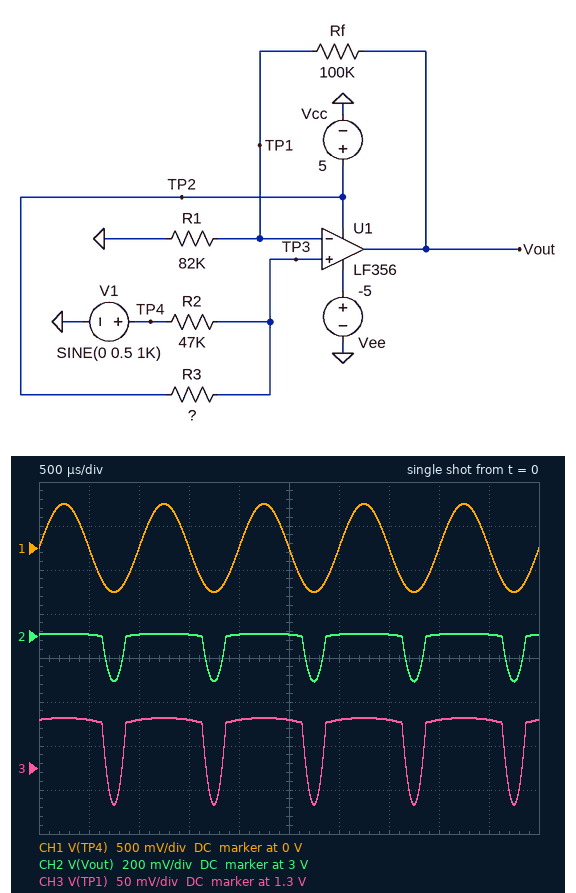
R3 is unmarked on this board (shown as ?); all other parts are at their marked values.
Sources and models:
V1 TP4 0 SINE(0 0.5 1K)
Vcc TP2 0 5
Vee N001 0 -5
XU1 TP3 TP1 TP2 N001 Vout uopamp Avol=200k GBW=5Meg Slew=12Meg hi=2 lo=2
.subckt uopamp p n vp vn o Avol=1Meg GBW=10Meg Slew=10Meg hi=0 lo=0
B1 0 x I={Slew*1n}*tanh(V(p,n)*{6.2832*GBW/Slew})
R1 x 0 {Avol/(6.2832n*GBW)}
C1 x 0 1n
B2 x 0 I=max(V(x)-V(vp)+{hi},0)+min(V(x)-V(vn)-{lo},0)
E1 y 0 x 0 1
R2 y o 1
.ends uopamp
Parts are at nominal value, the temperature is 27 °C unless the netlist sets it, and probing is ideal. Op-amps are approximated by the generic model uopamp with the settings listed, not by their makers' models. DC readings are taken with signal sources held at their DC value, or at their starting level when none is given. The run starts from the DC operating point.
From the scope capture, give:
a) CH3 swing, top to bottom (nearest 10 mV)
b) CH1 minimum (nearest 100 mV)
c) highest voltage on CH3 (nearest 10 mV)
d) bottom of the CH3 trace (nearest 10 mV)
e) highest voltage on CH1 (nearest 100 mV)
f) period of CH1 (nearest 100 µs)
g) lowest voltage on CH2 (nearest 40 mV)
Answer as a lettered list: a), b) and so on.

a) 100 mV
b) -500 mV
c) 1.36 V
d) 1.26 V
e) 500 mV
f) 1.0 ms
g) 2.80 V
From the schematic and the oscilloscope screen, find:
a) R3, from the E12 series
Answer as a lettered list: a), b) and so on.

a) 100 kΩ
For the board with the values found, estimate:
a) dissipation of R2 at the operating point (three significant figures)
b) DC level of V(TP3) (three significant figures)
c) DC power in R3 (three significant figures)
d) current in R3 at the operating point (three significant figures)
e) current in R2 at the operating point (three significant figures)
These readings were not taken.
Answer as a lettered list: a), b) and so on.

a) 54.4 µW
b) 1.60 V
c) 116 µW
d) 34.0 µA
e) 34.0 µA
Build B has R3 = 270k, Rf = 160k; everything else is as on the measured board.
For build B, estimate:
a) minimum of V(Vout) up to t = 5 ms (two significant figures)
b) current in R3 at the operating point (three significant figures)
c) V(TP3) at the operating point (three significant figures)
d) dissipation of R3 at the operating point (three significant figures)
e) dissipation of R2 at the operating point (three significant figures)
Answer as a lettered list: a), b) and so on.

a) 930 mV
b) 15.8 µA
c) 741 mV
d) 67.2 µW
e) 11.7 µW
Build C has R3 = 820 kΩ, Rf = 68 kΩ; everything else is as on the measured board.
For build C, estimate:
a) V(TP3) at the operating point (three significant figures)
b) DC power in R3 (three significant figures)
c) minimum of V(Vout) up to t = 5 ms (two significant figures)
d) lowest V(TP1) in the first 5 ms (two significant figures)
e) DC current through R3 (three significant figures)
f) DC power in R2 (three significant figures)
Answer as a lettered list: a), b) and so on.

a) 271 mV
b) 27.3 µW
c) -370 mV
d) -200 mV
e) 5.77 µA
f) 1.56 µW
